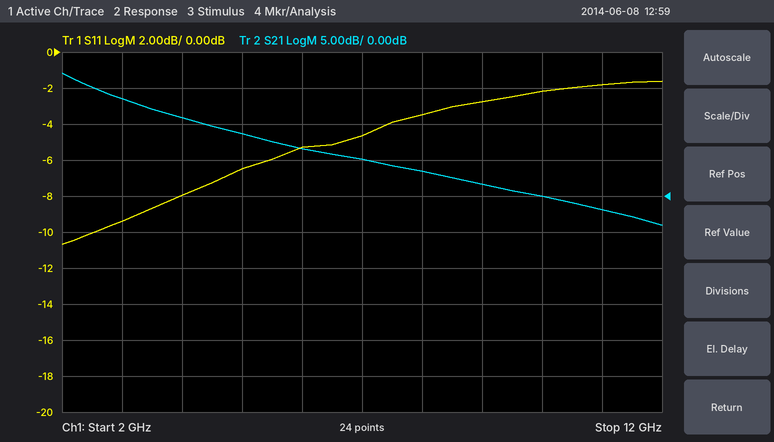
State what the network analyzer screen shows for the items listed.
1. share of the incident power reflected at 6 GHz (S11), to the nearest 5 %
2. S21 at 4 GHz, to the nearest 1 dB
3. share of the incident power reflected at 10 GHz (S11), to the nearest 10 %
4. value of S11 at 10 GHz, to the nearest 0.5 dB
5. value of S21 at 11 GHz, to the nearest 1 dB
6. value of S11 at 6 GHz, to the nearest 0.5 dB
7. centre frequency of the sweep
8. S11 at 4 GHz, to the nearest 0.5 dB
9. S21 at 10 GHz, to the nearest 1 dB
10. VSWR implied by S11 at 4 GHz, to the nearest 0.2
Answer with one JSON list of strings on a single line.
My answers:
["30 %", "11 dB", "60 %", "-2.0 dB", "-2 dB", "-5.5 dB", "7 GHz", "-8.0 dB", "0 dB", "2.4"]
